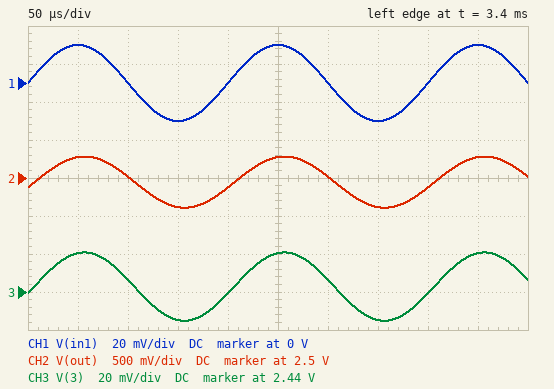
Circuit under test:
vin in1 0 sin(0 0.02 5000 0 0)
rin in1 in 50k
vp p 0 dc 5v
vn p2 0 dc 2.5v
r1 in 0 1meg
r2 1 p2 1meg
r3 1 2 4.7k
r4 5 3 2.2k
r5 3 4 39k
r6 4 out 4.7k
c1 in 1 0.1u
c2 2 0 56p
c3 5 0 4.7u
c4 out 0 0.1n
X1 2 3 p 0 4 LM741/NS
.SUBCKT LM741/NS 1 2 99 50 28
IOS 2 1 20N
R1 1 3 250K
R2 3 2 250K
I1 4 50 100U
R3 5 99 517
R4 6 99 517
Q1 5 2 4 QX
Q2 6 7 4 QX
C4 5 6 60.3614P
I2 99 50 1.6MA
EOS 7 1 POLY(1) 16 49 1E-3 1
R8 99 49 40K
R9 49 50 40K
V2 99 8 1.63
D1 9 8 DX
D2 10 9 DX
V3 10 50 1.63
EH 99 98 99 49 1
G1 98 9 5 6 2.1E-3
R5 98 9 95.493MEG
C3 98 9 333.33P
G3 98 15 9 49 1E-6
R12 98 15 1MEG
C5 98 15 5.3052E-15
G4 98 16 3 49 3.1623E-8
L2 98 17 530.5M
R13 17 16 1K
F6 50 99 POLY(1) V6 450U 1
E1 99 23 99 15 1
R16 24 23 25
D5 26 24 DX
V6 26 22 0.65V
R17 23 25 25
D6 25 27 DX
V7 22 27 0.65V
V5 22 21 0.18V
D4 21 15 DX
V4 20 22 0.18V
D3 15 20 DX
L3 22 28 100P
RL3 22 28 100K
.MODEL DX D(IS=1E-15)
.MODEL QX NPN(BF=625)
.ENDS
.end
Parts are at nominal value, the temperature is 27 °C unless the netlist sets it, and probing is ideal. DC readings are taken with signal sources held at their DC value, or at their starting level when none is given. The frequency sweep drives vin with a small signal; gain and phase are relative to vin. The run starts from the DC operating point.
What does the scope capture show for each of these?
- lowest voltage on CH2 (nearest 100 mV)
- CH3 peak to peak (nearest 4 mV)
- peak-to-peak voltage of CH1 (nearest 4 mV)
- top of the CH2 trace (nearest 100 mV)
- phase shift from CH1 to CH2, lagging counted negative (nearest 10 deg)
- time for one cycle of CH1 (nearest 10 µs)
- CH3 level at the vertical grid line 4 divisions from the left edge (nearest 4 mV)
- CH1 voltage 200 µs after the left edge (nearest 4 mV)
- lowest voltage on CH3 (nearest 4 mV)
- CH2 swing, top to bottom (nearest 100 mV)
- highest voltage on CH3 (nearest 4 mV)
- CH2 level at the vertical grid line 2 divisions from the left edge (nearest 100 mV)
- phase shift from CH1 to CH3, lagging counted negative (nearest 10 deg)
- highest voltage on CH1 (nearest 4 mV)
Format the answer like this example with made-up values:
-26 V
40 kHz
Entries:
2.1 V
36 mV
40 mV
2.8 V
-10 deg
200 µs
2.440 V
0 V
2.424 V
700 mV
2.460 V
2.5 V
-10 deg
20 mV
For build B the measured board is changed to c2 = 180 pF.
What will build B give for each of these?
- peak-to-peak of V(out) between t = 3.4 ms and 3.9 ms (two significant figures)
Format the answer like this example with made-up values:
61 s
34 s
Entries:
650 mV
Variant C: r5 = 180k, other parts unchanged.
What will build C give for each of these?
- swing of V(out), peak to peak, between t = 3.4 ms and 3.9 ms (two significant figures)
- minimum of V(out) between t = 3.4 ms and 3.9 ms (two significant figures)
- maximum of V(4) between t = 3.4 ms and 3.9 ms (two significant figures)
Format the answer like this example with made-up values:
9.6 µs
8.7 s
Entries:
2.7 V
1.1 V
3.8 V
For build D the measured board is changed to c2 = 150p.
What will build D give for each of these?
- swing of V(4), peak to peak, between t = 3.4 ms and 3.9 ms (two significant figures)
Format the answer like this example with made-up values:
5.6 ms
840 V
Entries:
660 mV
